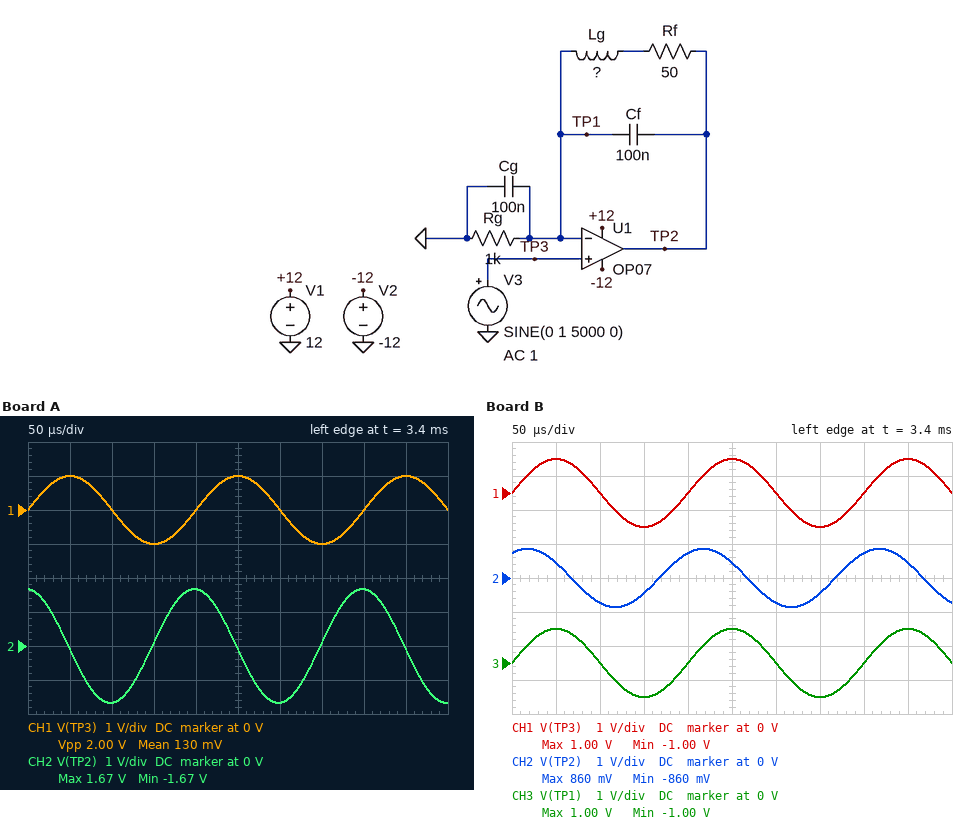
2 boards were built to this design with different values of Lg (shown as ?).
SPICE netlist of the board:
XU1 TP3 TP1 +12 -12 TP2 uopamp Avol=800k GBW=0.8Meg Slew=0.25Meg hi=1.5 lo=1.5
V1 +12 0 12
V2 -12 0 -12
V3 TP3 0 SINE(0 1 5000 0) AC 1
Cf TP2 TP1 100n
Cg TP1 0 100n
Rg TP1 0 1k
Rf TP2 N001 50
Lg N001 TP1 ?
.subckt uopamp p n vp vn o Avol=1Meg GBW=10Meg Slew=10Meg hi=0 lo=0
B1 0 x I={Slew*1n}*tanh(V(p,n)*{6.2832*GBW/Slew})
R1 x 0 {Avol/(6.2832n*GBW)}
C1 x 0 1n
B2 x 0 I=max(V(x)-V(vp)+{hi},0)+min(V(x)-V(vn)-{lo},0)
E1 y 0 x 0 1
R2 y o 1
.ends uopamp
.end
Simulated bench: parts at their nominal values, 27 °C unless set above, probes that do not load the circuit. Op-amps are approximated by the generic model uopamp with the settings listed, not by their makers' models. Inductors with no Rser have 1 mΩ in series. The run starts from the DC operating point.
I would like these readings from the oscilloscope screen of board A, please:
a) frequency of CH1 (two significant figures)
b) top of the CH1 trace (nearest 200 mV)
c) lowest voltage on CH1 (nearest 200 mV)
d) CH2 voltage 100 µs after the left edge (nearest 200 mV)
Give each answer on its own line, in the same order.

5.0 kHz
1.0 V
-1.0 V
-1.6 V
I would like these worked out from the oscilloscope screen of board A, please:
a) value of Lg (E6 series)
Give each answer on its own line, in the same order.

6.8 mH
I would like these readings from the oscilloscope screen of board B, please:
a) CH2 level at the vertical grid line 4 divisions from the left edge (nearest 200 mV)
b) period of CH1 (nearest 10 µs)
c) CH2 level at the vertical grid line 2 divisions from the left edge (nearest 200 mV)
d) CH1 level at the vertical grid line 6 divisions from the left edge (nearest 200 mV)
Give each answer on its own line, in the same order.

800 mV
200 µs
-800 mV
0 V
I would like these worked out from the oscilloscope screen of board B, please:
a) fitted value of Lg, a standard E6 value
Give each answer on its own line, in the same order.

4.7 mH
